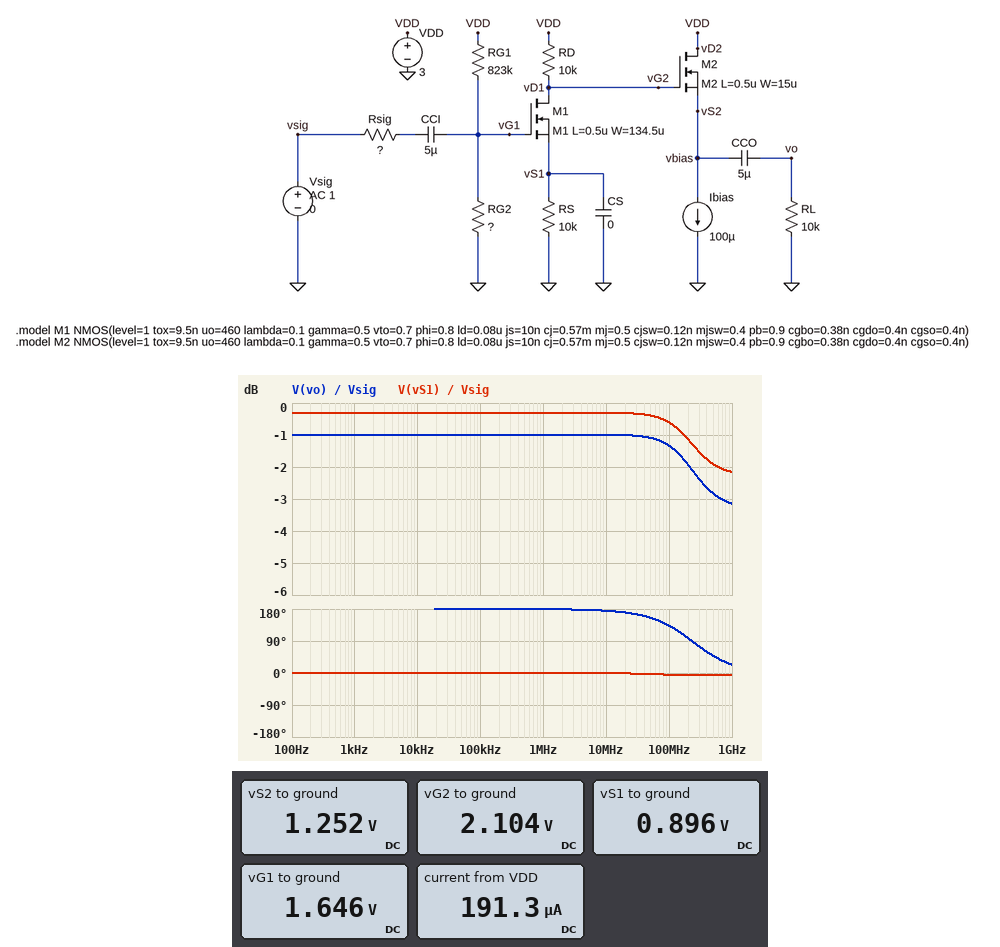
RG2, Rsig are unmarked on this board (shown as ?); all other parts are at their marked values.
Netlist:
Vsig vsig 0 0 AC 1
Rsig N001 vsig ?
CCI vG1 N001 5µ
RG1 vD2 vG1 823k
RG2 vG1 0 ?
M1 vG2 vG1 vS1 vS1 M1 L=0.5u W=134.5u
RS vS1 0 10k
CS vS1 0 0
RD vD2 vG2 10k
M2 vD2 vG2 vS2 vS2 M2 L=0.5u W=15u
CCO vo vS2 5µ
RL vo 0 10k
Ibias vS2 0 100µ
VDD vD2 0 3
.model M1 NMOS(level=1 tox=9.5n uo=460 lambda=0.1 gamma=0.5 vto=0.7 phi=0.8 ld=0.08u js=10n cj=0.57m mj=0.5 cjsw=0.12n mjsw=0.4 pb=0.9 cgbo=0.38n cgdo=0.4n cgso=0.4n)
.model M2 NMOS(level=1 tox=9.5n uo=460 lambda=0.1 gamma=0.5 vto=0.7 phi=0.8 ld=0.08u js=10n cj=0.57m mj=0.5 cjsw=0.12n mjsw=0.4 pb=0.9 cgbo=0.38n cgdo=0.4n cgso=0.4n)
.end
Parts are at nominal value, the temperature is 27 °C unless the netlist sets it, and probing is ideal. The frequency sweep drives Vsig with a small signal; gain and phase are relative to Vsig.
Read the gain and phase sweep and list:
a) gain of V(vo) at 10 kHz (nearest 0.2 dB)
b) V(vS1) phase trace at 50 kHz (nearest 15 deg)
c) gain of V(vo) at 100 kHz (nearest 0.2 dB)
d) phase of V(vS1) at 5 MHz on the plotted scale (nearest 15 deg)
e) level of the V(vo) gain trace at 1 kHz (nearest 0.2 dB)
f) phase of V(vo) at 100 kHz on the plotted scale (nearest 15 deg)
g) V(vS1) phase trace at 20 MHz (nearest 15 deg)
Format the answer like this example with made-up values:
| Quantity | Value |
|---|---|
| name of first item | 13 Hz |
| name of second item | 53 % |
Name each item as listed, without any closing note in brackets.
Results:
| Quantity | Value |
|---|---|
| gain of V(vo) at 10 kHz | -1.0 dB |
| V(vS1) phase trace at 50 kHz | 0 deg |
| gain of V(vo) at 100 kHz | -1.0 dB |
| phase of V(vS1) at 5 MHz on the plotted scale | 0 deg |
| level of the V(vo) gain trace at 1 kHz | -1.0 dB |
| phase of V(vo) at 100 kHz on the plotted scale | 180 deg |
| V(vS1) phase trace at 20 MHz | 0 deg |
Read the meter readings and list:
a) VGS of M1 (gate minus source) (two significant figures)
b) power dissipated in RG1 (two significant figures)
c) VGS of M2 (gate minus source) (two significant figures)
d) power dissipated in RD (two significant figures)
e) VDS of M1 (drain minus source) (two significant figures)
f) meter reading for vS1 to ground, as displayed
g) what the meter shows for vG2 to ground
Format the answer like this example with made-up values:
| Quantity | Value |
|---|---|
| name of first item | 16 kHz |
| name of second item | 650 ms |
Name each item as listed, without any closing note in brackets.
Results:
| Quantity | Value |
|---|---|
| VGS of M1 (gate minus source) | 750 mV |
| power dissipated in RG1 | 2.2 µW |
| VGS of M2 (gate minus source) | 850 mV |
| power dissipated in RD | 80 µW |
| VDS of M1 (drain minus source) | 1.2 V |
| meter reading for vS1 to ground, as displayed | 0.896 V |
| what the meter shows for vG2 to ground | 2.104 V |
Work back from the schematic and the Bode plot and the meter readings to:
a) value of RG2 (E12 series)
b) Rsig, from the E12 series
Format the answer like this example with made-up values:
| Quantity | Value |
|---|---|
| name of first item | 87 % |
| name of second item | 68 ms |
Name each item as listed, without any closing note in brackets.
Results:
| Quantity | Value |
|---|---|
| value of RG2 | 1 MΩ |
| Rsig, from the E12 series | 1.5 kΩ |
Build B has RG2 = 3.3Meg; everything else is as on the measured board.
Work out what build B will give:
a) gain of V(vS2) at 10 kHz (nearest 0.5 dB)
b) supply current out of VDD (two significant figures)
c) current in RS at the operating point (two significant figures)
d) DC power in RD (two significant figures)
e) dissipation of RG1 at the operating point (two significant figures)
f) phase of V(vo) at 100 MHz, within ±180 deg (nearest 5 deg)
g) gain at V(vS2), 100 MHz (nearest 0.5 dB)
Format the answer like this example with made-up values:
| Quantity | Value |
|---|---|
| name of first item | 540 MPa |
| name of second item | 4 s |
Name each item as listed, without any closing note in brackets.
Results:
| Quantity | Value |
|---|---|
| gain of V(vS2) at 10 kHz | -32.0 dB |
| supply current out of VDD | 250 µA |
| current in RS at the operating point | 150 µA |
| DC power in RD | 220 µW |
| dissipation of RG1 at the operating point | 440 nW |
| phase of V(vo) at 100 MHz, within ±180 deg | 45 deg |
| gain at V(vS2), 100 MHz | -5.5 dB |
